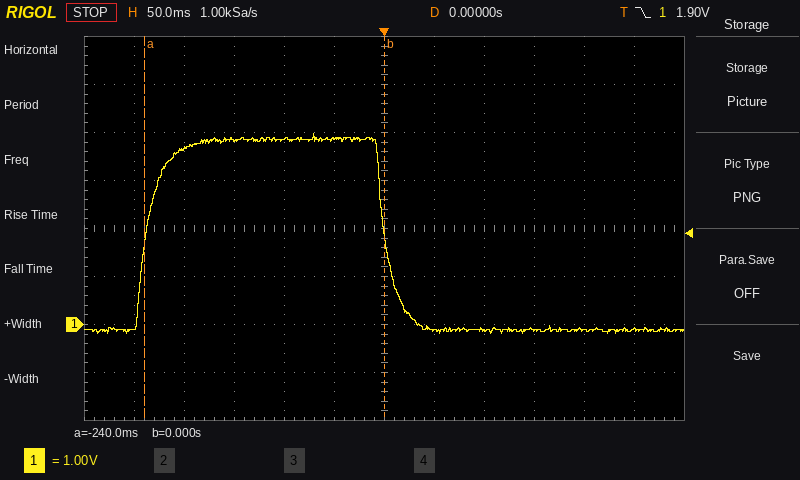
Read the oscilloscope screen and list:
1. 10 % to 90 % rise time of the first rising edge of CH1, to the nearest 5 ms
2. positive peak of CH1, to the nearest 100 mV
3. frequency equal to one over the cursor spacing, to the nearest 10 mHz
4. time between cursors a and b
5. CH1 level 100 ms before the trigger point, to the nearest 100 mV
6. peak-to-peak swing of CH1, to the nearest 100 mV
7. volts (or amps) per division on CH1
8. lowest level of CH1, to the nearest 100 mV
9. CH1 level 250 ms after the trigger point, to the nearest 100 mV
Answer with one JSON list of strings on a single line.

["35 ms", "4.0 V", "4.17 Hz", "240 ms", "3.9 V", "4.2 V", "1 V", "-200 mV", "-100 mV"]
